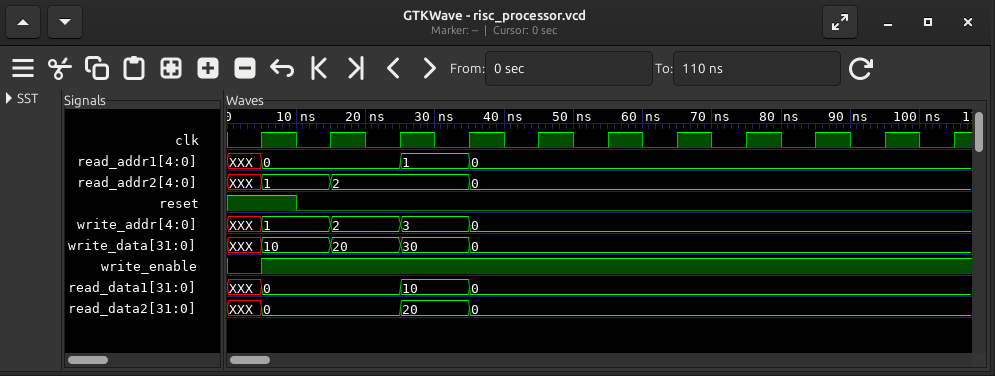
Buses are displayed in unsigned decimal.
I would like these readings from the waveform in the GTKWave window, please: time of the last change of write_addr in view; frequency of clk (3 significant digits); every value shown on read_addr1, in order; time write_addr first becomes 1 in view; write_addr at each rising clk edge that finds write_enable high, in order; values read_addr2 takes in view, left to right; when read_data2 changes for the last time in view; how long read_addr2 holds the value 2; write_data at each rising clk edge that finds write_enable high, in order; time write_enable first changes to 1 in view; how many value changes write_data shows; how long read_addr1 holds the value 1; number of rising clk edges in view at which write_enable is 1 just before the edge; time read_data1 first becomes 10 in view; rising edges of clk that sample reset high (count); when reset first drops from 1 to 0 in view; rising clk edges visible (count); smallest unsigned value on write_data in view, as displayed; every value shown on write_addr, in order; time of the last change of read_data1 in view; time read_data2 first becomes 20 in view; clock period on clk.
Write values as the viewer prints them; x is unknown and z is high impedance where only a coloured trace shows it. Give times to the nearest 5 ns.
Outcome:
35 ns
100 MHz
XXX, 0, 1, 0
5 ns
1, 2, 3, 0, 0, 0, 0, 0, 0, 0
XXX, 1, 2, 0
35 ns
20 ns
10, 20, 30, 0, 0, 0, 0, 0, 0, 0
5 ns
4
10 ns
10
25 ns
1
10 ns
11
0
XXX, 1, 2, 3, 0
35 ns
25 ns
10 ns
